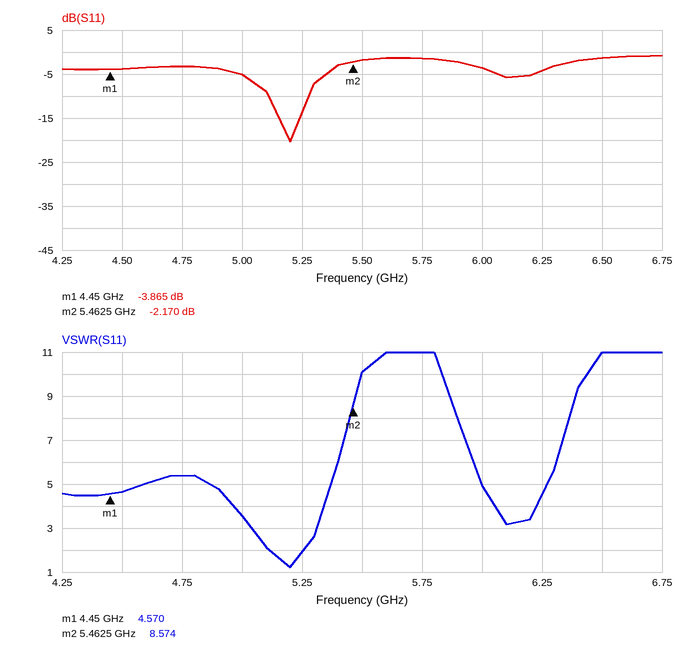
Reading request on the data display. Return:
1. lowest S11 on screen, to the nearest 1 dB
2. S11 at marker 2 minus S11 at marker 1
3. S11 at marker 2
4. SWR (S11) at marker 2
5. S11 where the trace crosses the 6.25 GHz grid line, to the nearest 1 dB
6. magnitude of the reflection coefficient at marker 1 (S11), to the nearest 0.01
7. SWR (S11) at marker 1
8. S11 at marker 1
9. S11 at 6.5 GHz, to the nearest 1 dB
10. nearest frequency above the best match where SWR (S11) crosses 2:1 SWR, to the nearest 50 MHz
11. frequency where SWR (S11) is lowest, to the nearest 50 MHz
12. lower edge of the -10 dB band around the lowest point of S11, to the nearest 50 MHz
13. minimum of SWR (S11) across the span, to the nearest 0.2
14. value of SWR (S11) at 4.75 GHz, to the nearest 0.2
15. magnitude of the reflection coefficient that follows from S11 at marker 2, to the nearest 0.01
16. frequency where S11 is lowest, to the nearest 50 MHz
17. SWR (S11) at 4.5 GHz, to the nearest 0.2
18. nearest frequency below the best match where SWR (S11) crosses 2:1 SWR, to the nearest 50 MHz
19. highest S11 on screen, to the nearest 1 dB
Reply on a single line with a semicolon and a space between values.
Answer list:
-20 dB; 1.695 dB; -2.170 dB; 8.574; -4 dB; 0.64; 4.570; -3.865 dB; -1 dB; 5.25 GHz; 5.20 GHz; 5.10 GHz; 1.2; 5.4; 0.78; 5.20 GHz; 4.6; 5.10 GHz; -1 dB
